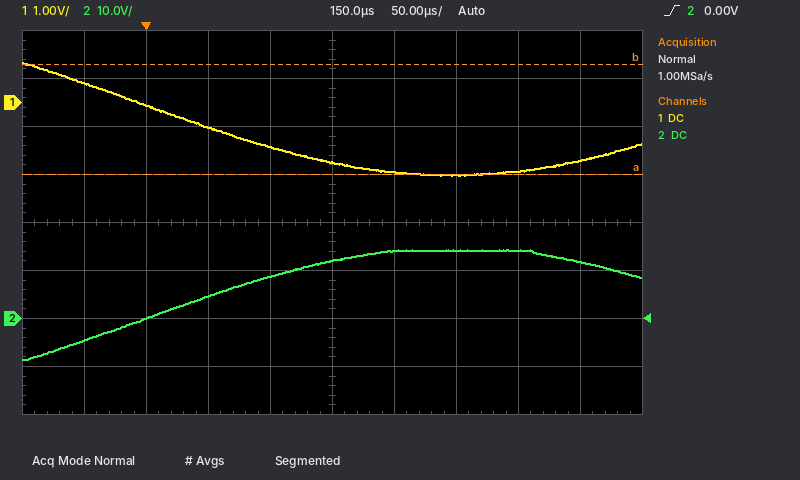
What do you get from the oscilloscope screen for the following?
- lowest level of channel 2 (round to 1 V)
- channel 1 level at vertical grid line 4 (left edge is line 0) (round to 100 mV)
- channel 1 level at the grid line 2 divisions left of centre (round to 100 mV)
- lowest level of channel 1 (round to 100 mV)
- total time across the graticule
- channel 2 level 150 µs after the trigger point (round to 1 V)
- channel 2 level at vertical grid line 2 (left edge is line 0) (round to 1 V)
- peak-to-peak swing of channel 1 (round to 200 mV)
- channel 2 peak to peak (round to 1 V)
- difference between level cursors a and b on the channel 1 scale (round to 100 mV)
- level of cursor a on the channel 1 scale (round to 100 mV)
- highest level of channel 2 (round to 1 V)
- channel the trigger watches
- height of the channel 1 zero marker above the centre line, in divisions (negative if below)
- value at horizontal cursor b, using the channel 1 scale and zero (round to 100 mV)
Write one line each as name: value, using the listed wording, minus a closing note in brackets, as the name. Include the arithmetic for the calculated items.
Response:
lowest level of channel 2: -9 V
channel 1 level at vertical grid line 4 (left edge is line 0): -900 mV
channel 1 level at the grid line 2 divisions left of centre: -500 mV
lowest level of channel 1: -1.5 V
total time across the graticule: 500 µs
channel 2 level 150 µs after the trigger point: 12 V
channel 2 level at vertical grid line 2 (left edge is line 0): 0 V
peak-to-peak swing of channel 1: 2.4 V
channel 2 peak to peak: 14 V − (-9 V) = 23 V
difference between level cursors a and b on the channel 1 scale: 2.3 V
level of cursor a on the channel 1 scale: -1.5 V
highest level of channel 2: 14 V
channel the trigger watches: channel 2
height of the channel 1 zero marker above the centre line, in divisions: +2.5 div
value at horizontal cursor b, using the channel 1 scale and zero: 800 mV
